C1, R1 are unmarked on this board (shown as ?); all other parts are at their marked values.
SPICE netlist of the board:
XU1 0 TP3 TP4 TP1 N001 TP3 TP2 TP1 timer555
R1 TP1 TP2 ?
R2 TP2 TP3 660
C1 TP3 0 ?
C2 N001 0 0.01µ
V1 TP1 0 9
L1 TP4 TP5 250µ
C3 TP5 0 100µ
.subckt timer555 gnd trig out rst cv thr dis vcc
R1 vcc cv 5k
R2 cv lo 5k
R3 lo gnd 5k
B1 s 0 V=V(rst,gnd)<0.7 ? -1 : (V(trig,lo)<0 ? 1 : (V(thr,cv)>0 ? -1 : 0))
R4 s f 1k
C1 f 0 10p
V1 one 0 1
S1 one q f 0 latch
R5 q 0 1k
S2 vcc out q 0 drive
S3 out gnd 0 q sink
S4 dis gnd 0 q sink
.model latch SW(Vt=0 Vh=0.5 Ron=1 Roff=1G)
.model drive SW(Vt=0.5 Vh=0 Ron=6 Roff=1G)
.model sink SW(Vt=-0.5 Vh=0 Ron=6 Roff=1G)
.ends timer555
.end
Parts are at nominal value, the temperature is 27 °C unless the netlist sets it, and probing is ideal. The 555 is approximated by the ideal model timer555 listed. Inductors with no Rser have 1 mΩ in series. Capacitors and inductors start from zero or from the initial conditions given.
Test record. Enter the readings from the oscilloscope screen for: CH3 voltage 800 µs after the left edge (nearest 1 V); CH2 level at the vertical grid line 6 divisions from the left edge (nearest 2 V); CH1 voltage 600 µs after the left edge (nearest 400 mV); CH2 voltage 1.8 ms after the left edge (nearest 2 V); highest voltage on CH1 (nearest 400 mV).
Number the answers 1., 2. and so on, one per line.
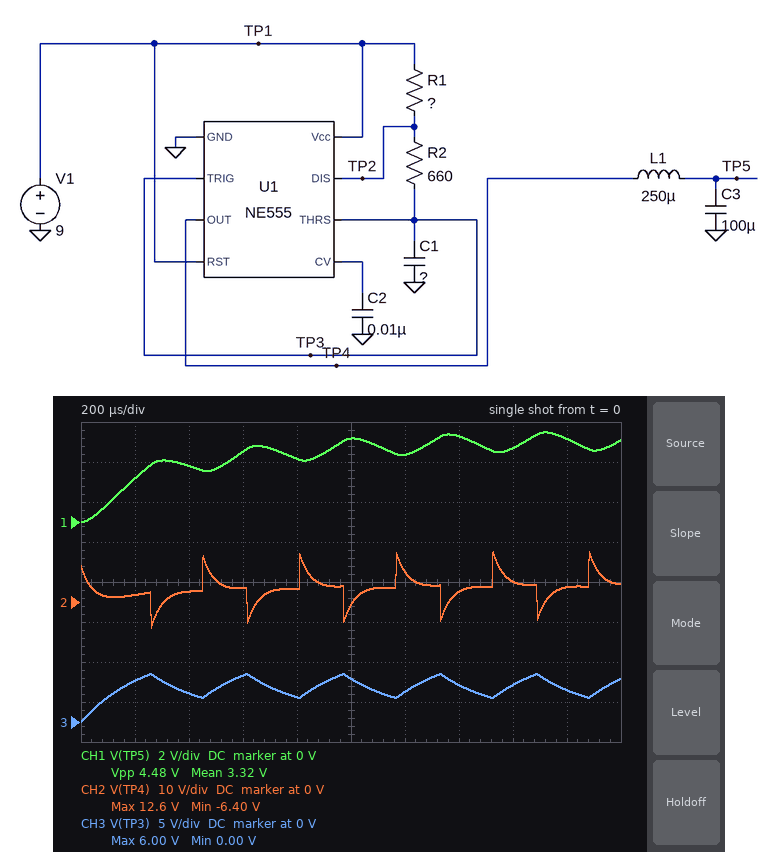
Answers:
1. 3 V
2. 8 V
3. 3.6 V
4. 4 V
5. 4.4 V
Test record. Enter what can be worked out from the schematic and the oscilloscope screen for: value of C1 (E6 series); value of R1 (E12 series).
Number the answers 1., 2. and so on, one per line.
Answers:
1. 330 nF
2. 56 Ω
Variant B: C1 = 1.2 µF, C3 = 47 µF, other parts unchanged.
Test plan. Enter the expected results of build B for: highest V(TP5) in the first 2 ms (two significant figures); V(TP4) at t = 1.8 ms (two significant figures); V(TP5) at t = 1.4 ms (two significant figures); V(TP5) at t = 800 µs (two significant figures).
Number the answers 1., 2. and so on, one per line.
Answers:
1. 8.8 V
2. 2.8 V
3. 1.6 V
4. 8.6 V
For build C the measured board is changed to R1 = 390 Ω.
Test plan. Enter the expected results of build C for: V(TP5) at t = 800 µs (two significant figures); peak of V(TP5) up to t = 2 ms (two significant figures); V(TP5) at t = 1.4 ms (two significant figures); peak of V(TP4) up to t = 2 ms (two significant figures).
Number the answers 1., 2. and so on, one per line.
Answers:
1. 5.1 V
2. 5.9 V
3. 4.7 V
4. 14 V
